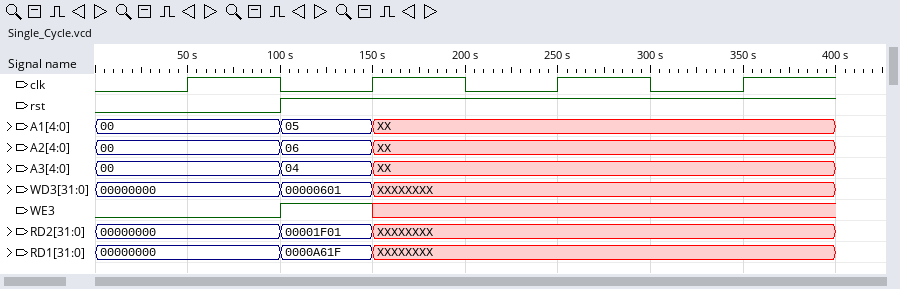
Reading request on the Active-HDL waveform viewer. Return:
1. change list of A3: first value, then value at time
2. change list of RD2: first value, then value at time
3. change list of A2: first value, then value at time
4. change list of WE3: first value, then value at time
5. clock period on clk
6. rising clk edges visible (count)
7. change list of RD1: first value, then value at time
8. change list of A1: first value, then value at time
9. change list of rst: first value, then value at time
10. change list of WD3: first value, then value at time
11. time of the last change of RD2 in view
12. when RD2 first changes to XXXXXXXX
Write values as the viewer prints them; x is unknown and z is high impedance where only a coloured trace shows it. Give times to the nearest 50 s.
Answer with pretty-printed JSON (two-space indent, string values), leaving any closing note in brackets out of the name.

{
  "change list of A3: first value, then value at time": "00, 04 at 100 s, XX at 150 s",
  "change list of RD2: first value, then value at time": "00000000, 00001F01 at 100 s, XXXXXXXX at 150 s",
  "change list of A2: first value, then value at time": "00, 06 at 100 s, XX at 150 s",
  "change list of WE3: first value, then value at time": "0, 1 at 100 s, x at 150 s",
  "clock period on clk": "100 s",
  "rising clk edges visible": "4",
  "change list of RD1: first value, then value at time": "00000000, 0000A61F at 100 s, XXXXXXXX at 150 s",
  "change list of A1: first value, then value at time": "00, 05 at 100 s, XX at 150 s",
  "change list of rst: first value, then value at time": "0, 1 at 100 s",
  "change list of WD3: first value, then value at time": "00000000, 00000601 at 100 s, XXXXXXXX at 150 s",
  "time of the last change of RD2 in view": "150 s",
  "when RD2 first changes to XXXXXXXX": "150 s"
}
